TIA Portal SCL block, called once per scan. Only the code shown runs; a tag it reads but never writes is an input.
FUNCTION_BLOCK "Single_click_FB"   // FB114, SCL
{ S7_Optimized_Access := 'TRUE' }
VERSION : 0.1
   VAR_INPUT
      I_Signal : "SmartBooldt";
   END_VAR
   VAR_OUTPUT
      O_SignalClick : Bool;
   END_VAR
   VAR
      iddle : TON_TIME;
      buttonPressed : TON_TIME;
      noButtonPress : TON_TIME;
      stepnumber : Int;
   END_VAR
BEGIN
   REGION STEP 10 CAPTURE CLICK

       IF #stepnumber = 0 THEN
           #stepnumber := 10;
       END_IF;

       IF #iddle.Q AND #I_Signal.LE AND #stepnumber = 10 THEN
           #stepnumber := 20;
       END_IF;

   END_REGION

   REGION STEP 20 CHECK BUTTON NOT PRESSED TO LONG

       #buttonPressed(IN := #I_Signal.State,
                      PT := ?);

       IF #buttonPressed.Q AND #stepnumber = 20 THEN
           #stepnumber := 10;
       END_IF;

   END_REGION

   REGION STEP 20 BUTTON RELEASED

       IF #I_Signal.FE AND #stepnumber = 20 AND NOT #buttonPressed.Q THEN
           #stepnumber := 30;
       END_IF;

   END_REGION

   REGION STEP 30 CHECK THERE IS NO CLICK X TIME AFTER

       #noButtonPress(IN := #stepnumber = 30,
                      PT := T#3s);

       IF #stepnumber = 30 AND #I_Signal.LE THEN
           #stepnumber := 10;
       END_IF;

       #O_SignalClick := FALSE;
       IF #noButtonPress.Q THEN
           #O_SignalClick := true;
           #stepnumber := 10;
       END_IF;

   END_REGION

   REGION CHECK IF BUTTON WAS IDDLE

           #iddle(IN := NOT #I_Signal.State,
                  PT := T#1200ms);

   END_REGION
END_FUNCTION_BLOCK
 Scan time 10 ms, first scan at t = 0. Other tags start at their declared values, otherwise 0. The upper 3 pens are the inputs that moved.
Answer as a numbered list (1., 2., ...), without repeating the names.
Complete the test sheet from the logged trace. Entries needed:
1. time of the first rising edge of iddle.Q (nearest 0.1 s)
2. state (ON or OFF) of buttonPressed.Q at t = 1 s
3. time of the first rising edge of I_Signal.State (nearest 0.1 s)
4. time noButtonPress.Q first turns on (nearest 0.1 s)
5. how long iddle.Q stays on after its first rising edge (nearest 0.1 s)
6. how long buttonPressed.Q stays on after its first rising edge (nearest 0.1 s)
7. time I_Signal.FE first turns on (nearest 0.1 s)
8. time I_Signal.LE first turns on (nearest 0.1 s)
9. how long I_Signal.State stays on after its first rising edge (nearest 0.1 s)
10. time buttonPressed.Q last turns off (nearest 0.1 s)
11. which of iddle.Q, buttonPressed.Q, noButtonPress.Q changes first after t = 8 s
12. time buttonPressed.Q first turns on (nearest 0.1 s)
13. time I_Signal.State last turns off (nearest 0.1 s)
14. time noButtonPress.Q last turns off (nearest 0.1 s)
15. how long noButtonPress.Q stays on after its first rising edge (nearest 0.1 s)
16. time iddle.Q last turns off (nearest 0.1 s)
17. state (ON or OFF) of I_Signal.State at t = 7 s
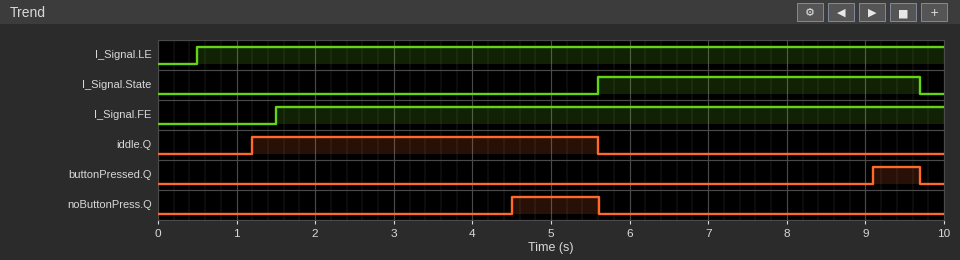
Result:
1. 1.2 s
2. OFF
3. 5.6 s
4. 4.5 s
5. 4.4 s
6. 0.6 s
7. 1.5 s
8. 0.5 s
9. 4.1 s
10. 9.7 s
11. buttonPressed.Q
12. 9.1 s
13. 9.7 s
14. 5.6 s
15. 1.1 s
16. 5.6 s
17. ON
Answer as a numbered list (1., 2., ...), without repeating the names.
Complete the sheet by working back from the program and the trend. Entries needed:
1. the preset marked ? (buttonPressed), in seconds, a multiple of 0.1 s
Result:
1. 3.5 s
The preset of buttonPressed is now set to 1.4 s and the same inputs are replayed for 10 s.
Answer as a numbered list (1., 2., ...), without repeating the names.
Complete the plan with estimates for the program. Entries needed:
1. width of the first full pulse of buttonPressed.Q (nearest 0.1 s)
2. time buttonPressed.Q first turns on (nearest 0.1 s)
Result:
1. 2.7 s
2. 7.0 s
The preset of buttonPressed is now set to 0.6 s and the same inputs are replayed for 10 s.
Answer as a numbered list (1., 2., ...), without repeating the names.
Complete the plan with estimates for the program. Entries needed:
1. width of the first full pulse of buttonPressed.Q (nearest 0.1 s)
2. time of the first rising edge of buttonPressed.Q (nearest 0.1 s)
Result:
1. 3.5 s
2. 6.2 s
